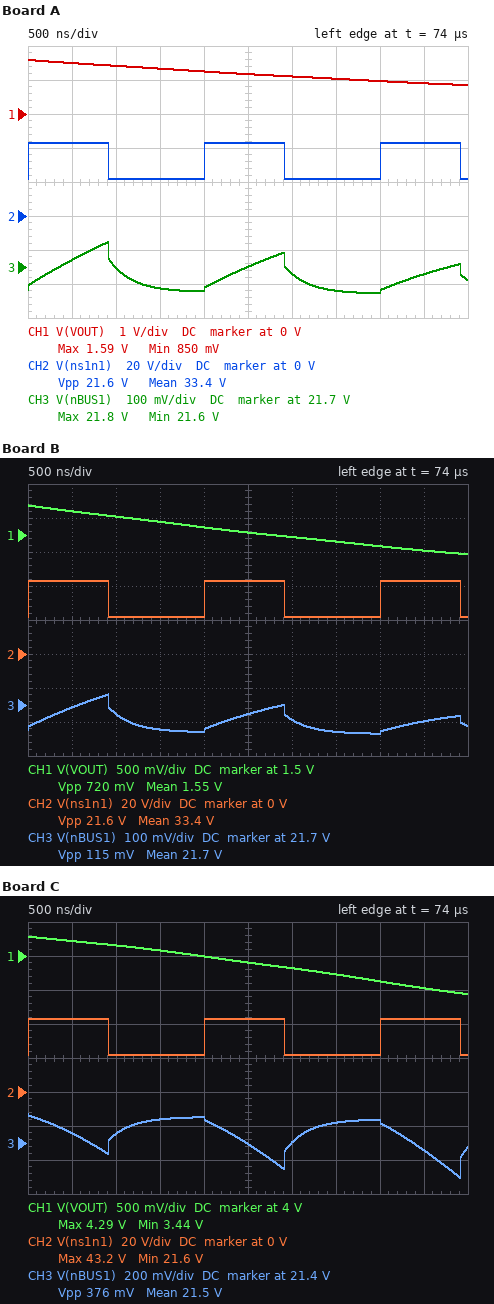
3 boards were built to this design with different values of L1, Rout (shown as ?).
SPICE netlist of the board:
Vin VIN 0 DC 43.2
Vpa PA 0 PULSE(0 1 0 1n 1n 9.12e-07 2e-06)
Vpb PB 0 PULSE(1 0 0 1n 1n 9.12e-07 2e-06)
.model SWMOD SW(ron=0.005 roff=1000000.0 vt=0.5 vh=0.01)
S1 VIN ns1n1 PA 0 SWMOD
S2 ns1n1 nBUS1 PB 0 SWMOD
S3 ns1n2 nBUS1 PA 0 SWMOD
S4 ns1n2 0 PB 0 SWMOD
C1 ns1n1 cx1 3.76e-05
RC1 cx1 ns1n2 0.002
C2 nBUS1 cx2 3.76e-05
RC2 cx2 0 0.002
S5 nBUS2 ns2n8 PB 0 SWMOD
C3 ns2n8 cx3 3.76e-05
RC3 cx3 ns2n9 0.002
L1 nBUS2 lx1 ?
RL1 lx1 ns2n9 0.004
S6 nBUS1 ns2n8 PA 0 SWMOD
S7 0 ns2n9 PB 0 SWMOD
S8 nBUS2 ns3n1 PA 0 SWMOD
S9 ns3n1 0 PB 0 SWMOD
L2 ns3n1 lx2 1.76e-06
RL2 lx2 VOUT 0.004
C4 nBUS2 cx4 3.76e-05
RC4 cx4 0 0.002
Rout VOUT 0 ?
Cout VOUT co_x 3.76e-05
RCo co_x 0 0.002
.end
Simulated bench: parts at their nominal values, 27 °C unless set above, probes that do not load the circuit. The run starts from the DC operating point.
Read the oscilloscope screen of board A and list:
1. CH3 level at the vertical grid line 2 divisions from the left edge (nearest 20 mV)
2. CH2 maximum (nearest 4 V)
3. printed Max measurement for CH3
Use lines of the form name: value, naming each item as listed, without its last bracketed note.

CH3 level at the vertical grid line 2 divisions from the left edge: 21.70 V
CH2 maximum: 44 V
printed Max measurement for CH3: 21.8 V
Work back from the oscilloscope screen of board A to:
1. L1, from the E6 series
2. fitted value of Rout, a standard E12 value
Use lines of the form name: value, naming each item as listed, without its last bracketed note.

L1, from the E6 series: 4.7 µH
fitted value of Rout, a standard E12 value: 0.56 Ω
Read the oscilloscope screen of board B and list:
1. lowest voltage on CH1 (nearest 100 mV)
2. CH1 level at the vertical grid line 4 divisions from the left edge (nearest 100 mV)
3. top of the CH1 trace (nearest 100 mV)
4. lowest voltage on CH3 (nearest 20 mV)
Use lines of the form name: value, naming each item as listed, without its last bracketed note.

lowest voltage on CH1: 1.2 V
CH1 level at the vertical grid line 4 divisions from the left edge: 1.6 V
top of the CH1 trace: 1.9 V
lowest voltage on CH3: 21.62 V
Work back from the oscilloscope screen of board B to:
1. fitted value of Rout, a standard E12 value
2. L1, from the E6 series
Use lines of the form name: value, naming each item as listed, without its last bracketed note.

fitted value of Rout, a standard E12 value: 0.39 Ω
L1, from the E6 series: 4.7 µH
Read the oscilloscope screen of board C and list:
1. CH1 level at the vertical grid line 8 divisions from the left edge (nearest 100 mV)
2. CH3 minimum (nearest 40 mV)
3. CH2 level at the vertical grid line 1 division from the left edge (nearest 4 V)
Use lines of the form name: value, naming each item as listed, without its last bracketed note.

CH1 level at the vertical grid line 8 divisions from the left edge: 3.6 V
CH3 minimum: 21.20 V
CH2 level at the vertical grid line 1 division from the left edge: 44 V
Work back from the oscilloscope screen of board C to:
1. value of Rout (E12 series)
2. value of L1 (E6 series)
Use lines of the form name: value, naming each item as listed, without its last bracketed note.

value of Rout: 0.56 Ω
value of L1: 1 µH
